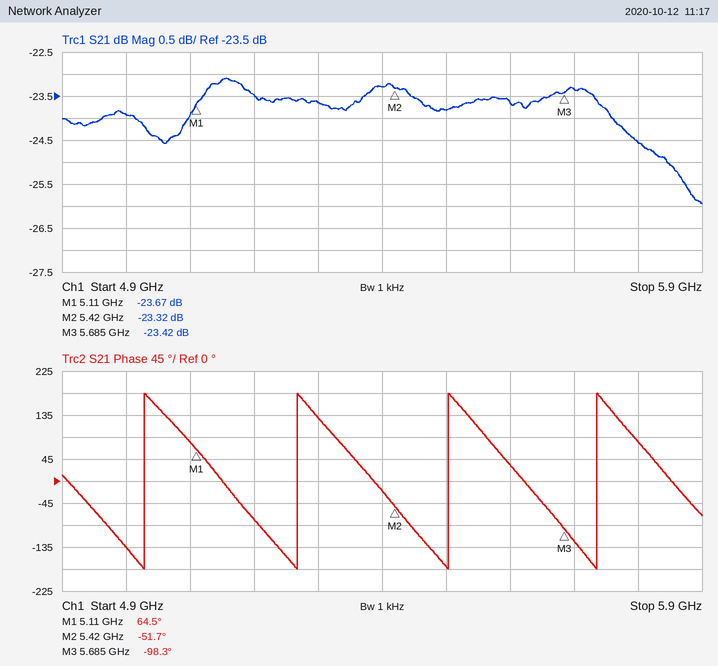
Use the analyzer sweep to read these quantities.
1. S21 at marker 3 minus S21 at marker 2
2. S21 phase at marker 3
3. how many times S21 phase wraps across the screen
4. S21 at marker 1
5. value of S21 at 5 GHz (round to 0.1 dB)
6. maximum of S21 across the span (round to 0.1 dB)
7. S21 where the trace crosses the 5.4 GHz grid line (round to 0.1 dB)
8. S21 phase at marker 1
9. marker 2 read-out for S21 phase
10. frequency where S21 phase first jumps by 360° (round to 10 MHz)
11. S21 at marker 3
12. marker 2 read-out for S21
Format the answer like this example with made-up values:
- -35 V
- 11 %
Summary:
- -0.10 dB
- -98.3°
- 4
- -23.67 dB
- -23.9 dB
- -23.1 dB
- -23.3 dB
- 64.5°
- -51.7°
- 5.03 GHz
- -23.42 dB
- -23.32 dB
